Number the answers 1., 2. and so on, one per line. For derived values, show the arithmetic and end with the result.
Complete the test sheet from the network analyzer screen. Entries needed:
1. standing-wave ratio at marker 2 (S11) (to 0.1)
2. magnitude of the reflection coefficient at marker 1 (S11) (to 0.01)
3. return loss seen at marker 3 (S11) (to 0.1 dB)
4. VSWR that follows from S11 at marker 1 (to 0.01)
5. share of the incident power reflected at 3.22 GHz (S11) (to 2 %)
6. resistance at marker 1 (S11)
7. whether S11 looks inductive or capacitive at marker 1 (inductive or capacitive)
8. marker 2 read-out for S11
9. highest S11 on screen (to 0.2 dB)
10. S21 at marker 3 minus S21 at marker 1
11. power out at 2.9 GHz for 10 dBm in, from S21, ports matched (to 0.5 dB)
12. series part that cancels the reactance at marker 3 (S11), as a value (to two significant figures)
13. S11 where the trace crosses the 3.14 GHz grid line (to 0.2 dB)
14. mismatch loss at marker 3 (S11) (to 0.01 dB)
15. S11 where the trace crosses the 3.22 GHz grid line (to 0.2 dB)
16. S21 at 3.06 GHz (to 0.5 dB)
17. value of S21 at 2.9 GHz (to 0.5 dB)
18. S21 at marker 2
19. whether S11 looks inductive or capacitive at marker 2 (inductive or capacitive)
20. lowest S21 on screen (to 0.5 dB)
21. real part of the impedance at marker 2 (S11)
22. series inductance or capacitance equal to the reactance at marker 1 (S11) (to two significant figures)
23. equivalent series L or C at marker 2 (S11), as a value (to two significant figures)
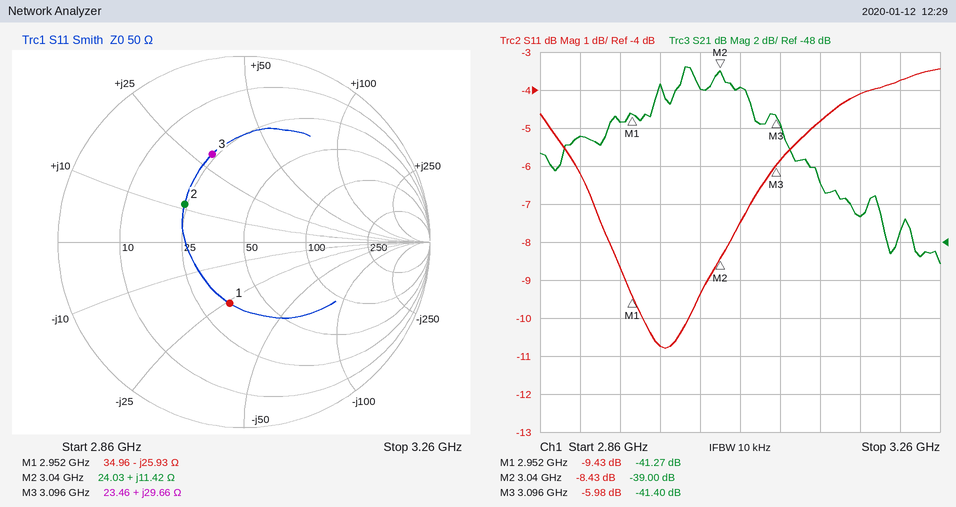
1. 2.2
2. 0.34
3. 6.0 dB
4. (1 + 0.3377)/(1 − 0.3377) ≈ 2.02
5. 10^(-3.8/10) ≈ 42 %
6. 34.96 Ω
7. capacitive
8. -8.43 dB
9. -3.4 dB
10. -41.4 − (-41.27) = -0.13 dB
11. 10 dBm + (-42.5 dB) = -32.5 dBm
12. C = 1/(2π × 3.096 GHz × 29.66 Ω) ≈ 1.7 pF
13. -4.8 dB
14. −10 log10(1 − 10^(-5.98/10)) ≈ 1.26 dB
15. -3.8 dB
16. -40.0 dB
17. -42.5 dB
18. -39.00 dB
19. inductive
20. -49.0 dB
21. 24.03 Ω
22. C = 1/(2π × 2.952 GHz × 25.93 Ω) ≈ 2.1 pF
23. L = 11.42 Ω/(2π × 3.04 GHz) ≈ 598 pH, so 600 pH to two significant figures
